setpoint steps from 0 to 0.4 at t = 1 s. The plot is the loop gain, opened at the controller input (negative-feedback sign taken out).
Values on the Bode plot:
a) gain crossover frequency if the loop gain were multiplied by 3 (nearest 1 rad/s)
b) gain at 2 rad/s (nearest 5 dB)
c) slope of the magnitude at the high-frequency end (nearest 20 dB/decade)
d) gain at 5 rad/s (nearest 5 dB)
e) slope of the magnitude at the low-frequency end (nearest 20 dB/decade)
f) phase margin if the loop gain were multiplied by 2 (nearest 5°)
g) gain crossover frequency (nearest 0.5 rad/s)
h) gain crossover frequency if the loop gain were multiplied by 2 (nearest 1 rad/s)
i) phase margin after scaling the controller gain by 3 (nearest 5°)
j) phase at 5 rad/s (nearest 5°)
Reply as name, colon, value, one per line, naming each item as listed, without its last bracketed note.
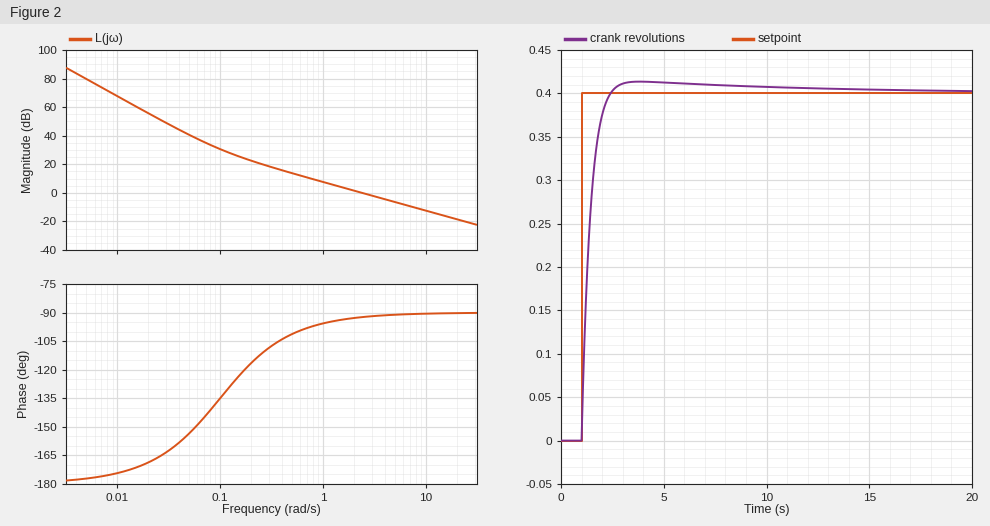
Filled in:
gain crossover frequency if the loop gain were multiplied by 3: 7 rad/s
gain at 2 rad/s: 0 dB
slope of the magnitude at the high-frequency end: -20 dB/decade
gain at 5 rad/s: -5 dB
slope of the magnitude at the low-frequency end: -40 dB/decade
phase margin if the loop gain were multiplied by 2: 90°
gain crossover frequency: 2.5 rad/s
gain crossover frequency if the loop gain were multiplied by 2: 5 rad/s
phase margin after scaling the controller gain by 3: 90°
phase at 5 rad/s: -90°
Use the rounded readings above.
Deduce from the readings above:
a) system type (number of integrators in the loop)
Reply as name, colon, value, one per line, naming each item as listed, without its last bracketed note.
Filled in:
system type: 2
